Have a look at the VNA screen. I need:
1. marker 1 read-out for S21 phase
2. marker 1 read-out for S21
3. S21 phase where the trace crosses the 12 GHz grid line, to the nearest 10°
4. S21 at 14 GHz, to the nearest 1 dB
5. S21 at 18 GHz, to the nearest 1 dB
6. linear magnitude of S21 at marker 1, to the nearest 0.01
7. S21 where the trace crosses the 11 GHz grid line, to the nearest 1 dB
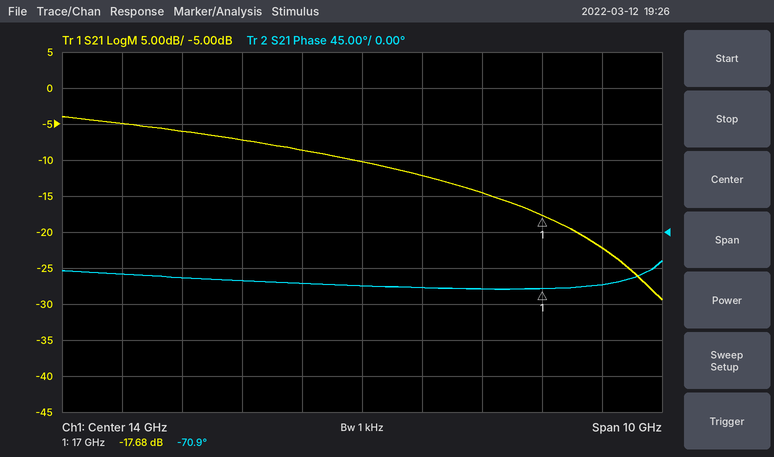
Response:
-70.9°
-17.68 dB
-60°
-10 dB
-22 dB
0.13
-6 dB
